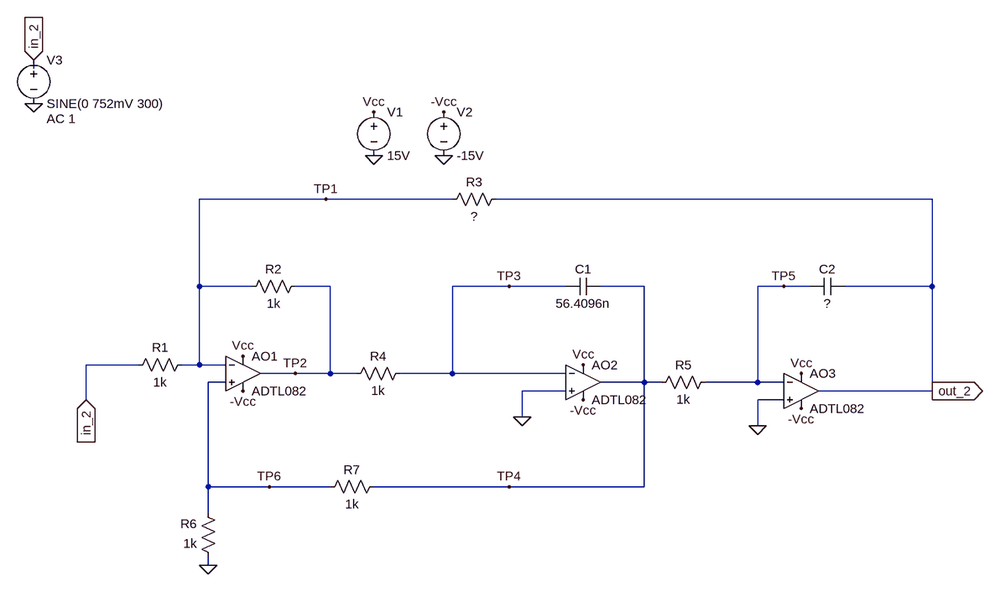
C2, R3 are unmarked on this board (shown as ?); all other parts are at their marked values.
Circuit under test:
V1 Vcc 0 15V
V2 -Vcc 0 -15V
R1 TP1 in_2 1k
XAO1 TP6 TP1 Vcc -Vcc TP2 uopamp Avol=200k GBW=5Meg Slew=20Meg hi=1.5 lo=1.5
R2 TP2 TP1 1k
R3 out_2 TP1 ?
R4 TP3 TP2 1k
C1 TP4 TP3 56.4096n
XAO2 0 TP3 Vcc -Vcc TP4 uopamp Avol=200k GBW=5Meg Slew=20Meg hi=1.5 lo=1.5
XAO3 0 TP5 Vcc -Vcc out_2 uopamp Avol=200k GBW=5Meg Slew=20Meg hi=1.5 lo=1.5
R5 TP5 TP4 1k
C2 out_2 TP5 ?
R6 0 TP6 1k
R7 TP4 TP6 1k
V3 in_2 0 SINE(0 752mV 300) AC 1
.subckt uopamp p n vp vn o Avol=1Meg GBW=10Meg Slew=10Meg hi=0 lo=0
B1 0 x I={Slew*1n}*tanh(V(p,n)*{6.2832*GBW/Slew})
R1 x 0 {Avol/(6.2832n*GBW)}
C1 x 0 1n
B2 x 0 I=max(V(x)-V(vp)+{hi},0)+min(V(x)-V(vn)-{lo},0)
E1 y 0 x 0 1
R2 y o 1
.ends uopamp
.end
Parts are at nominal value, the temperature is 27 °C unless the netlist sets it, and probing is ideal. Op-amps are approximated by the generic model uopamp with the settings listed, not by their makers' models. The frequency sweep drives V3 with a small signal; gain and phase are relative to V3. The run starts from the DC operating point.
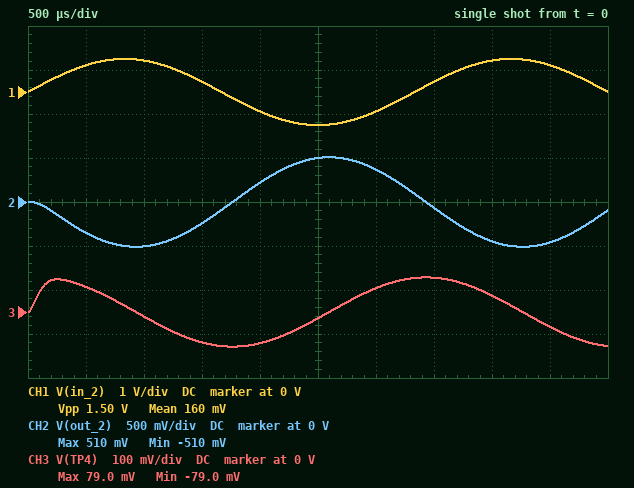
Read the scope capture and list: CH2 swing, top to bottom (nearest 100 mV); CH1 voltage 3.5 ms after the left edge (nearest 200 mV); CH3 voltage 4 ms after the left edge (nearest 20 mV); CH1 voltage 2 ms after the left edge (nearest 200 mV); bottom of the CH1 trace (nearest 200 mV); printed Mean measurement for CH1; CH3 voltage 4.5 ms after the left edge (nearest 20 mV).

1.0 V
200 mV
40 mV
-400 mV
-800 mV
160 mV
-40 mV
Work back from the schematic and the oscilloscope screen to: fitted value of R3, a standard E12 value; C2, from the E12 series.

680 Ω
82 nF
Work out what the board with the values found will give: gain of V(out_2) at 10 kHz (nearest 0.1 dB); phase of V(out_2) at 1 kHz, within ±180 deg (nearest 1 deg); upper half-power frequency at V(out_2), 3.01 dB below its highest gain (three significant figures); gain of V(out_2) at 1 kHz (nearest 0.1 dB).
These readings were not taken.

-25.6 dB
145 deg
2.25 kHz
-3.9 dB
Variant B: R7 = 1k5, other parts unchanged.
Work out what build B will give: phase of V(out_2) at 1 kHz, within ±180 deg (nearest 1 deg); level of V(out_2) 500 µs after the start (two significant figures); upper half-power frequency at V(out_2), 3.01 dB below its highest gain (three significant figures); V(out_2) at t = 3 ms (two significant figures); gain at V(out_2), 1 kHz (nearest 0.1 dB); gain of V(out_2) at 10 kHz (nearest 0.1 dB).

151 deg
-370 mV
2.91 kHz
360 mV
-3.4 dB
-25.2 dB
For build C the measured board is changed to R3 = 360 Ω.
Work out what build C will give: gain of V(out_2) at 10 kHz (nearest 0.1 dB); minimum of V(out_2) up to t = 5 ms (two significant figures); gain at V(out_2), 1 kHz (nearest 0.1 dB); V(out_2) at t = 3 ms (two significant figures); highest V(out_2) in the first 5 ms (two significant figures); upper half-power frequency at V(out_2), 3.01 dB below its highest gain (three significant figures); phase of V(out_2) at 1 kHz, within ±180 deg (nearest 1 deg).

-25.9 dB
-270 mV
-9.2 dB
190 mV
270 mV
3.08 kHz
155 deg
